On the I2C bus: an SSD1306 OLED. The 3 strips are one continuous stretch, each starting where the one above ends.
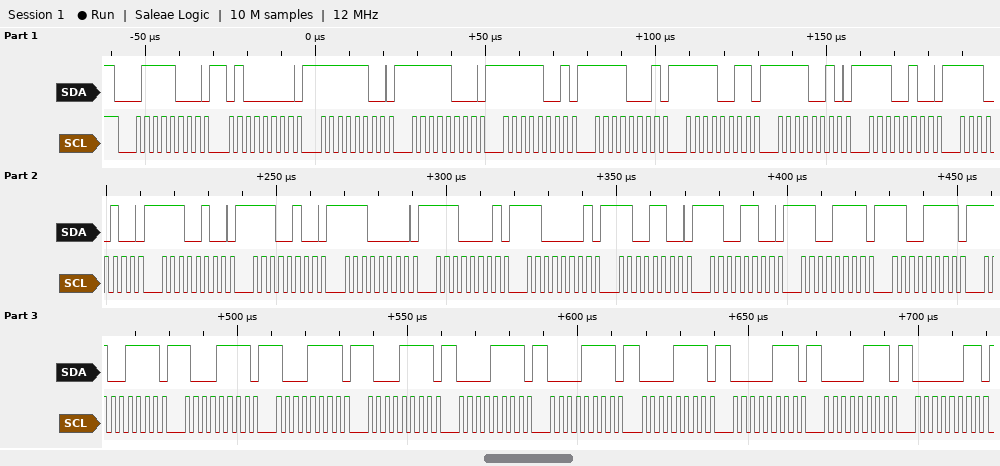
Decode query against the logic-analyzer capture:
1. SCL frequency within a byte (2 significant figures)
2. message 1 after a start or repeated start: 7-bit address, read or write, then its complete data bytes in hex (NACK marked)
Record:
400 kHz
0x3C write: 40 FC F8 F9 F1 F3 F2 E4 E4 E4 E4 E0 E1 C1 CC CC CF CF CF 8F 8F 8F 0F 0F 0F 07 07 03
